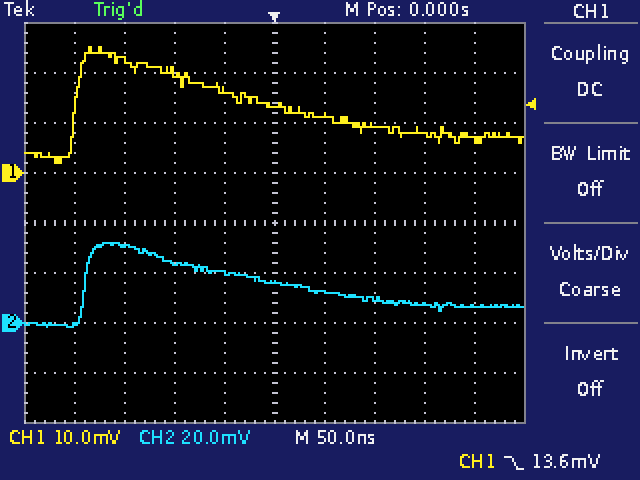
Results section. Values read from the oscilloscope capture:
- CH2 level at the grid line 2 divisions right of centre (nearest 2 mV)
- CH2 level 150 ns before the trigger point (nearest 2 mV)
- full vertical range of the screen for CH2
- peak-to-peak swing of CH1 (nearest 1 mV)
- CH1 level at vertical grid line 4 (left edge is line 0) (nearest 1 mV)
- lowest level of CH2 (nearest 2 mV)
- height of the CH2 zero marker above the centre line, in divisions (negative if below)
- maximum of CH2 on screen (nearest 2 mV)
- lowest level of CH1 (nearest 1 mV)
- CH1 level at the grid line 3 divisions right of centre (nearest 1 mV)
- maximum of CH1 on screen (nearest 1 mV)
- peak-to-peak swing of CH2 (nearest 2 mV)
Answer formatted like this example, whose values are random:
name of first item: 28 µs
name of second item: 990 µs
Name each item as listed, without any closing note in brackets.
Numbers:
CH2 level at the grid line 2 divisions right of centre: 10 mV
CH2 level 150 ns before the trigger point: 30 mV
full vertical range of the screen for CH2: 160 mV
peak-to-peak swing of CH1: 23 mV
CH1 level at vertical grid line 4 (left edge is line 0): 17 mV
lowest level of CH2: -2 mV
height of the CH2 zero marker above the centre line, in divisions: -2.0 div
maximum of CH2 on screen: 32 mV
lowest level of CH1: 2 mV
CH1 level at the grid line 3 divisions right of centre: 8 mV
maximum of CH1 on screen: 25 mV
peak-to-peak swing of CH2: 34 mV
